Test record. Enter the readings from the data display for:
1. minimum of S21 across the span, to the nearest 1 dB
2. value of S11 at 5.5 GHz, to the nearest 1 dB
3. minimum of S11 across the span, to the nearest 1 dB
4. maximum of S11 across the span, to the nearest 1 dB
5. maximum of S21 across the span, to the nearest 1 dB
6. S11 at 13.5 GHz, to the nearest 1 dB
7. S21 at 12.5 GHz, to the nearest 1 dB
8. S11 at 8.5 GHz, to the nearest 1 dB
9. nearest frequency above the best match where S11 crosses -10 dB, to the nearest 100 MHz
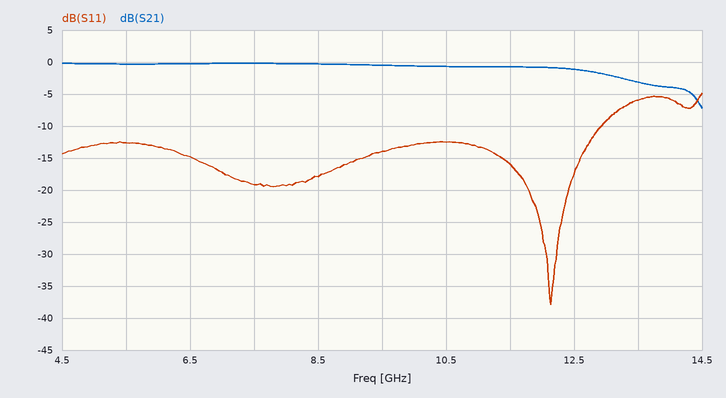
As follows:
-7 dB
-13 dB
-38 dB
-5 dB
0 dB
-6 dB
-1 dB
-18 dB
12.9 GHz
